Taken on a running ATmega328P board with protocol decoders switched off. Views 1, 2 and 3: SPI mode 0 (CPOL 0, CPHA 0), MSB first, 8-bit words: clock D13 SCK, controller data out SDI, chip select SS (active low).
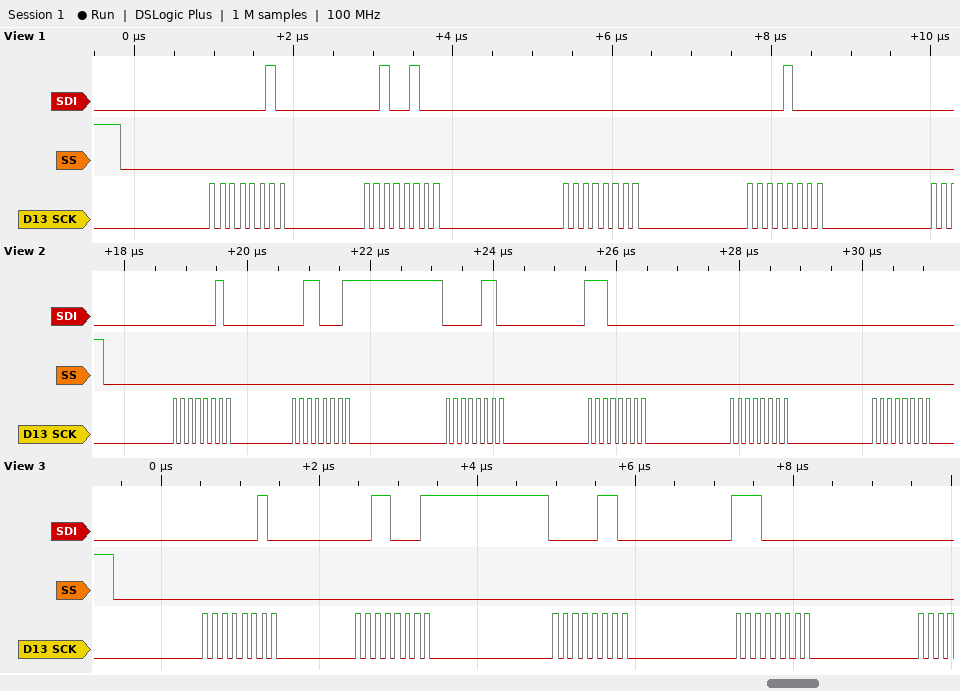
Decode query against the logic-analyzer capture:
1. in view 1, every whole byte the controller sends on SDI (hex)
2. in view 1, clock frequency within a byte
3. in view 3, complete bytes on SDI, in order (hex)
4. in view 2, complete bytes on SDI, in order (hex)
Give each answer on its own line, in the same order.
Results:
02 24 00 08
8 MHz
0x02 0x31 0x06 0xE0
02 31 06 E0 00 00
